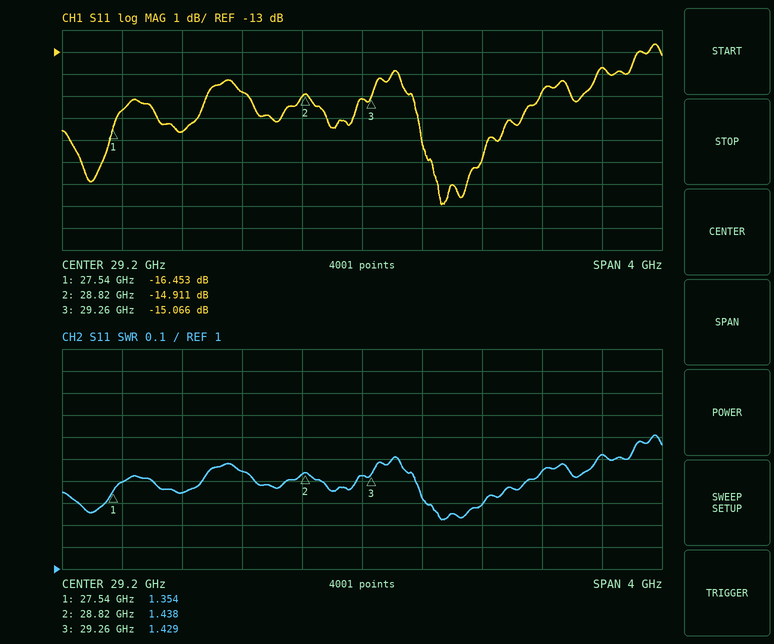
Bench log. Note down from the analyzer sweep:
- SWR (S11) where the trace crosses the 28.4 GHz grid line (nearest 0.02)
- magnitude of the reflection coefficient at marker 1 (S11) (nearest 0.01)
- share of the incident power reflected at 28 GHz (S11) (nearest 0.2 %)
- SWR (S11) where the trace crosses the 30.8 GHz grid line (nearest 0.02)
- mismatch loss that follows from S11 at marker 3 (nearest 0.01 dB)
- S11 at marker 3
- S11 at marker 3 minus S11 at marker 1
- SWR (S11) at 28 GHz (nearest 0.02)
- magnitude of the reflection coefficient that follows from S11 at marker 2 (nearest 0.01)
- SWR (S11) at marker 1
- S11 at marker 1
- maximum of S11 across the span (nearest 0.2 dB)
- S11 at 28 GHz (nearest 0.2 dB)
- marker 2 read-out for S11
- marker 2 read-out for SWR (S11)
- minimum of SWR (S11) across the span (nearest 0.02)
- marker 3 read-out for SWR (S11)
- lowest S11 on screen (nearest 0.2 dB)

1.44
0.15
2.2 %
1.52
0.14 dB
-15.066 dB
1.387 dB
1.34
0.18
1.354
-16.453 dB
-12.6 dB
-16.6 dB
-14.911 dB
1.438
1.22
1.429
-20.0 dB
